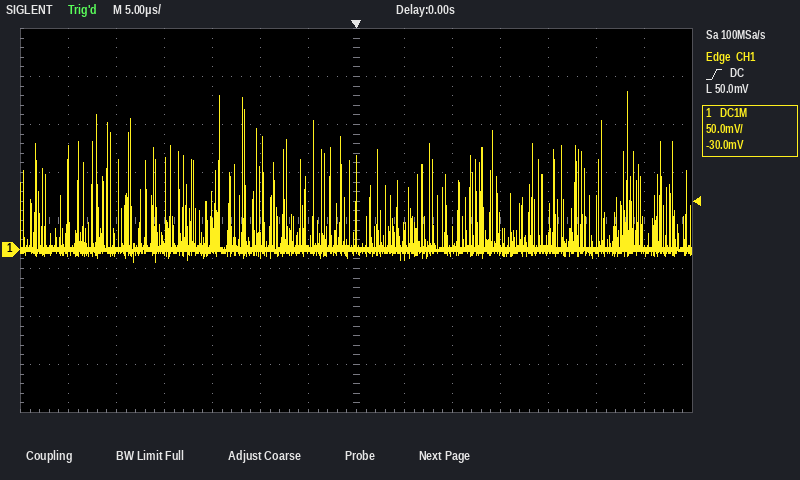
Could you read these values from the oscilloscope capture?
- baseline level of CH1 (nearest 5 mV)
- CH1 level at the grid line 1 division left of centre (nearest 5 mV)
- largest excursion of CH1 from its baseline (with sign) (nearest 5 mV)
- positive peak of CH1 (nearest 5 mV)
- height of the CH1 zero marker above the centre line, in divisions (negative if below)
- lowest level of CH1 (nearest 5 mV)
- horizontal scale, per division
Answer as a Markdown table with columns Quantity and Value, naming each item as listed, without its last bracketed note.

| Quantity | Value |
|---|---|
| baseline level of CH1 | 0 mV |
| CH1 level at the grid line 1 division left of centre | 0 mV |
| largest excursion of CH1 from its baseline (with sign) | +165 mV |
| positive peak of CH1 | 165 mV |
| height of the CH1 zero marker above the centre line, in divisions | -0.6 div |
| lowest level of CH1 | -15 mV |
| horizontal scale, per division | 5 µs |
